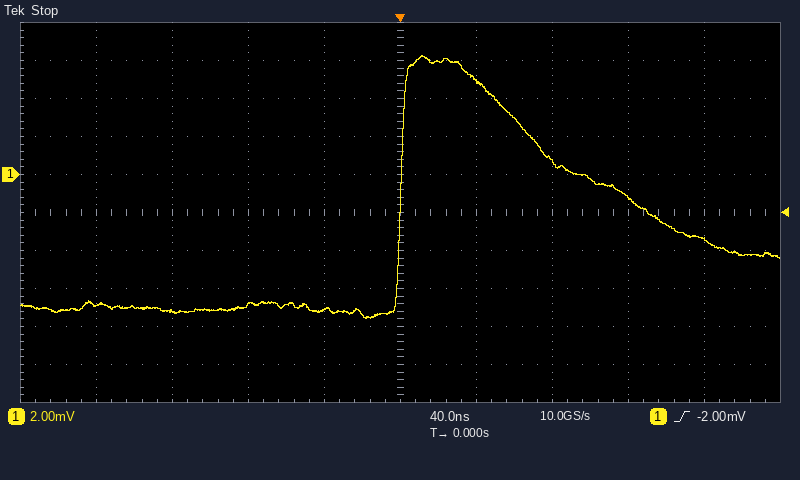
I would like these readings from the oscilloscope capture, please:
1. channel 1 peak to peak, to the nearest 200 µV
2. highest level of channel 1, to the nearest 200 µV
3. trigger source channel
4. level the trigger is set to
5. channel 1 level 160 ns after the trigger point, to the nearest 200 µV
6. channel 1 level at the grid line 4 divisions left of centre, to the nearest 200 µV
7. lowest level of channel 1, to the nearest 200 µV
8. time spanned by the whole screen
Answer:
13.8 mV
6.2 mV
channel 1
-2.00 mV
-3.4 mV
-6.8 mV
-7.6 mV
400 ns
